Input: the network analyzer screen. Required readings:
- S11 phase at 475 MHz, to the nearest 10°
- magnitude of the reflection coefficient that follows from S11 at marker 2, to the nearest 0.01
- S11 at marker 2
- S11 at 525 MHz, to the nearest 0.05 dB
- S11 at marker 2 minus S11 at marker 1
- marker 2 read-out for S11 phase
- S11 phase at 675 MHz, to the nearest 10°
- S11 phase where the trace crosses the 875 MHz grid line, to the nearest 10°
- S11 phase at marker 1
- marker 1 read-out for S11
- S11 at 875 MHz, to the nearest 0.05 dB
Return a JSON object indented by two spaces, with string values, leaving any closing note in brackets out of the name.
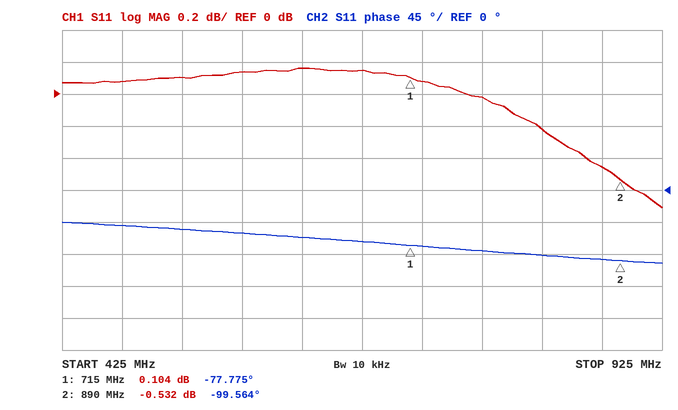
{
  "S11 phase at 475 MHz, to the nearest 10°": "-50°",
  "magnitude of the reflection coefficient that follows from S11 at marker 2, to the nearest 0.01": "0.94",
  "S11 at marker 2": "-0.532 dB",
  "S11 at 525 MHz, to the nearest 0.05 dB": "0.10 dB",
  "S11 at marker 2 minus S11 at marker 1": "-0.636 dB",
  "marker 2 read-out for S11 phase": "-99.564°",
  "S11 phase at 675 MHz, to the nearest 10°": "-70°",
  "S11 phase where the trace crosses the 875 MHz grid line, to the nearest 10°": "-100°",
  "S11 phase at marker 1": "-77.775°",
  "marker 1 read-out for S11": "0.104 dB",
  "S11 at 875 MHz, to the nearest 0.05 dB": "-0.45 dB"
}
